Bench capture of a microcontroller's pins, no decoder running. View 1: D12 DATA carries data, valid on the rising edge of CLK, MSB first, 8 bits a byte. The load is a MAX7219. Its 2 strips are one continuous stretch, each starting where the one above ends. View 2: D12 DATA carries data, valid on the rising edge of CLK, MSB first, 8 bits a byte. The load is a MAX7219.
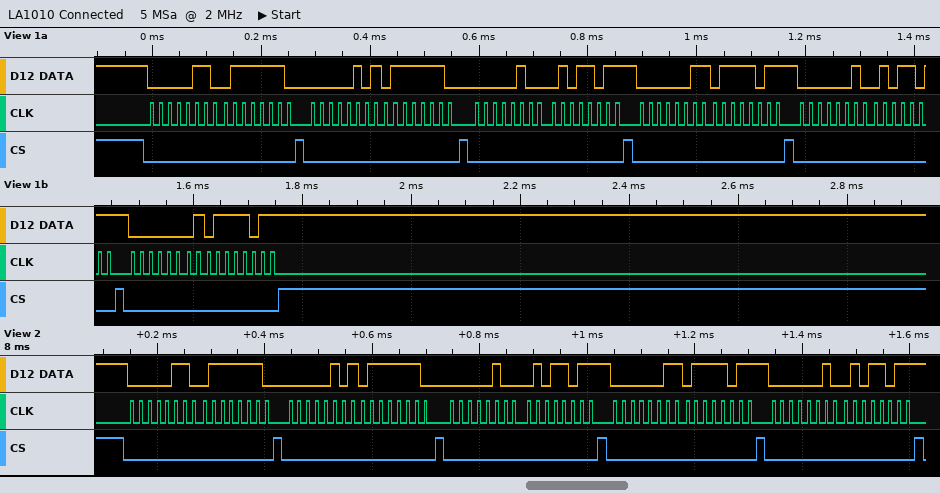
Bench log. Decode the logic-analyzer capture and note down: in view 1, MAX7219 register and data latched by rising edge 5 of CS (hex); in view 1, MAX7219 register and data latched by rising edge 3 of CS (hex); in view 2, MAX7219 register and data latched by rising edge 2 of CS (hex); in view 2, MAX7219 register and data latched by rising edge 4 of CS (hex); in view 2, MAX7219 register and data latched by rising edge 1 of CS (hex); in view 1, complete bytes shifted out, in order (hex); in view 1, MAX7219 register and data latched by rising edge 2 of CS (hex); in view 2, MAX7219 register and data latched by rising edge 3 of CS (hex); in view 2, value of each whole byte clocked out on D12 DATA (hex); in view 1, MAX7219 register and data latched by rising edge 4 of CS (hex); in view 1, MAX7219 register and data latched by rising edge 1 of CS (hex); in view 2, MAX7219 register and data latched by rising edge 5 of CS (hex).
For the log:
register 0x2, data 0x5B
register 0x4, data 0x5B
register 0x5, data 0x7E
register 0x3, data 0x7B
register 0x6, data 0x7E
06 7E 05 7E 04 5B 03 7B 02 5B 01 7B
register 0x5, data 0x7E
register 0x4, data 0x5B
06 7E 05 7E 04 5B 03 7B 02 5B
register 0x3, data 0x7B
register 0x6, data 0x7E
register 0x2, data 0x5B
